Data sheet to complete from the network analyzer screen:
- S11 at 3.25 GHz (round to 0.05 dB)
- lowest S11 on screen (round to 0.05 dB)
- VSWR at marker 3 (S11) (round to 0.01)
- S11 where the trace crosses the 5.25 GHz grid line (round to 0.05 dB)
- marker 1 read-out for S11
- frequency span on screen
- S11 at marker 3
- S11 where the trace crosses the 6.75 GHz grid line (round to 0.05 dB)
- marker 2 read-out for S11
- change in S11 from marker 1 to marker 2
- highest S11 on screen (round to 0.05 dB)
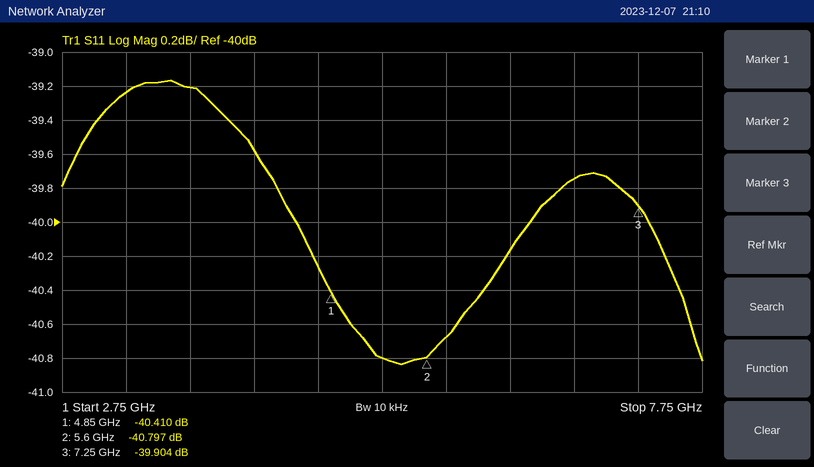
-39.25 dB
-40.85 dB
1.02
-40.80 dB
-40.410 dB
5 GHz
-39.904 dB
-39.75 dB
-40.797 dB
-0.387 dB
-39.15 dB
